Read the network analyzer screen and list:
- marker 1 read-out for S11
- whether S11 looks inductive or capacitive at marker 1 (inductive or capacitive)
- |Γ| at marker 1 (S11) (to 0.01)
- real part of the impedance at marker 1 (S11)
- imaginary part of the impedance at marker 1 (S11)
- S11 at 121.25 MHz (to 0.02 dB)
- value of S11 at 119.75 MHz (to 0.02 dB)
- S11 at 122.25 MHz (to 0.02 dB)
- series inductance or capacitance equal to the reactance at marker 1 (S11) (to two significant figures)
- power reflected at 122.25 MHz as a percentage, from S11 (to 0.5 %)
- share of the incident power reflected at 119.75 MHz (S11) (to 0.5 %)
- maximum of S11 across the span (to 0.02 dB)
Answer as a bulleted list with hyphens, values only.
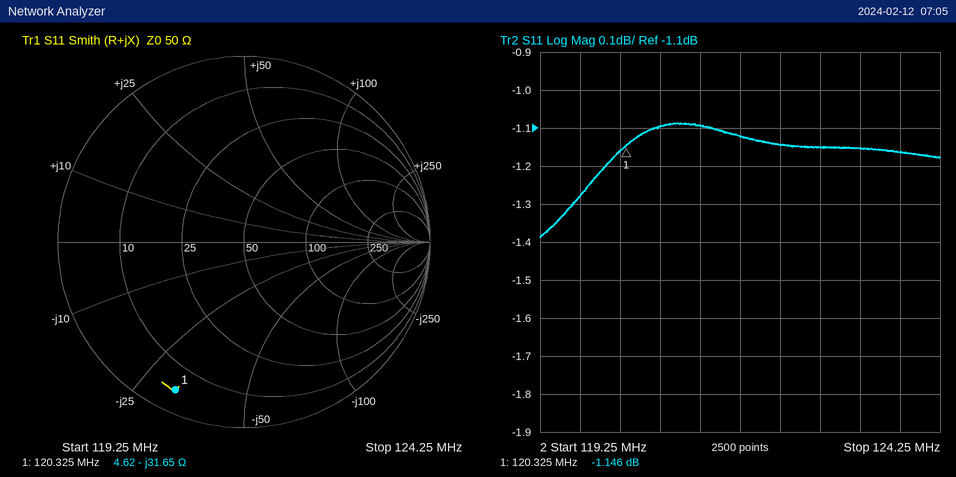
- -1.146 dB
- capacitive
- 0.88
- 4.62 Ω
- -31.65 Ω
- -1.10 dB
- -1.28 dB
- -1.14 dB
- 42 pF
- 77.0 %
- 74.5 %
- -1.08 dB
